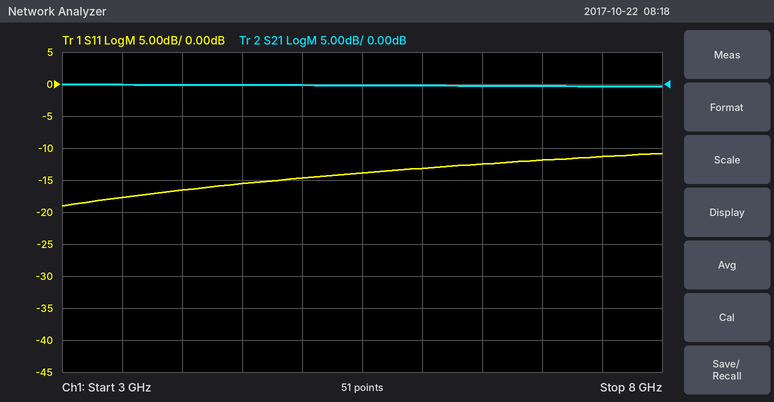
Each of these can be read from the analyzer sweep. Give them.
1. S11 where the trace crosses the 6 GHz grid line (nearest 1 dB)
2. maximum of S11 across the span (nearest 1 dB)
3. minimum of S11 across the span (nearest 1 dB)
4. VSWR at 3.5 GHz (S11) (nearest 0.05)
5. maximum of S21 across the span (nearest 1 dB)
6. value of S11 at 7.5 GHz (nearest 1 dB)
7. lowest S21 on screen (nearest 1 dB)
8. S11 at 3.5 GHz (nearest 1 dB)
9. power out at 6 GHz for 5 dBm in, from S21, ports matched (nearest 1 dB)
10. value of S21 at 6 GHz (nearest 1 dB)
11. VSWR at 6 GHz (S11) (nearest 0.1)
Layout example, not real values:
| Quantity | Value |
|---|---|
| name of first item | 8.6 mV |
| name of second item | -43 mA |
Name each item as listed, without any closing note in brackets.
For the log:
| Quantity | Value |
|---|---|
| S11 where the trace crosses the 6 GHz grid line | -13 dB |
| maximum of S11 across the span | -11 dB |
| minimum of S11 across the span | -19 dB |
| VSWR at 3.5 GHz (S11) | 1.30 |
| maximum of S21 across the span | 0 dB |
| value of S11 at 7.5 GHz | -11 dB |
| lowest S21 on screen | 0 dB |
| S11 at 3.5 GHz | -18 dB |
| power out at 6 GHz for 5 dBm in, from S21, ports matched | 5 dBm |
| value of S21 at 6 GHz | 0 dB |
| VSWR at 6 GHz (S11) | 1.6 |
